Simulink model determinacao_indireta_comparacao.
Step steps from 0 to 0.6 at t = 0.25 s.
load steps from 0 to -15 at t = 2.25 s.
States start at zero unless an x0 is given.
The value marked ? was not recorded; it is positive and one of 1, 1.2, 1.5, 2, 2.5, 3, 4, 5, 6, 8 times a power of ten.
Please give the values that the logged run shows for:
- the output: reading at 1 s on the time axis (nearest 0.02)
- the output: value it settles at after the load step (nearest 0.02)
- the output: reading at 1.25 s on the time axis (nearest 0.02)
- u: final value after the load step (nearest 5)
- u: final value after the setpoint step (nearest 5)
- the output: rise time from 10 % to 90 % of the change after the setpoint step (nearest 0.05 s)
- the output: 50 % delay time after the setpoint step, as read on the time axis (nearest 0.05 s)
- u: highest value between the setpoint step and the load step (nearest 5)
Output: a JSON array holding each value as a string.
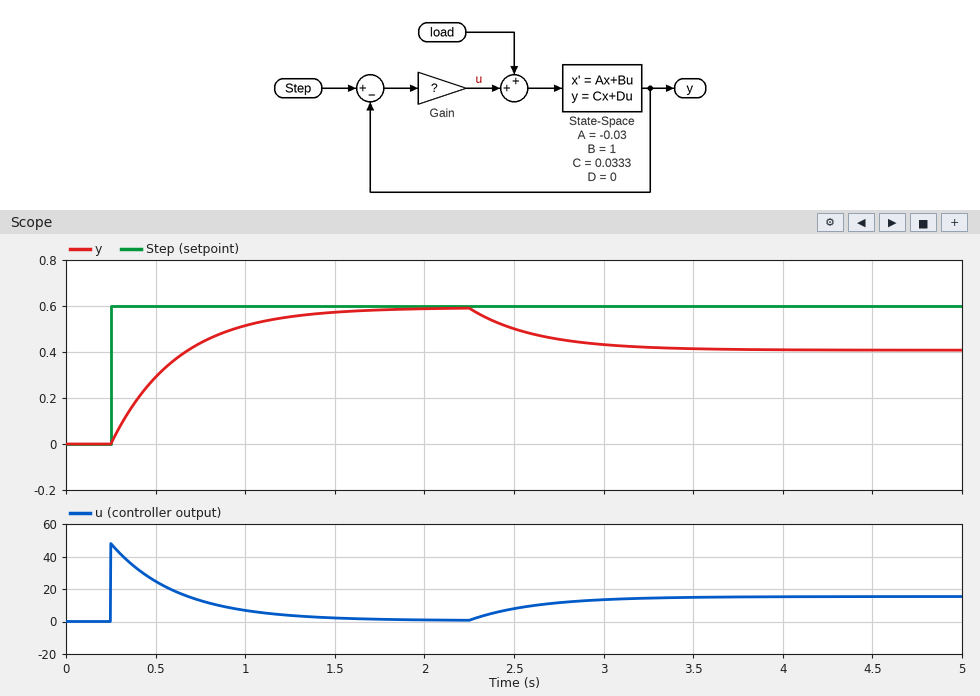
["0.52", "0.40", "0.56", "15", "0", "0.80 s", "0.50 s", "50"]
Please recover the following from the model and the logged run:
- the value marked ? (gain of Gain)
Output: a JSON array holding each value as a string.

["80"]
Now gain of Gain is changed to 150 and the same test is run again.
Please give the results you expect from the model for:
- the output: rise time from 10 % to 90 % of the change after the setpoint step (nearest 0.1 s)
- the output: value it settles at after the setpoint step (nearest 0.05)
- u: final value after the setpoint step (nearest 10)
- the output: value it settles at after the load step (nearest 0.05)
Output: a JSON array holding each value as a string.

["0.4 s", "0.60", "0", "0.50"]
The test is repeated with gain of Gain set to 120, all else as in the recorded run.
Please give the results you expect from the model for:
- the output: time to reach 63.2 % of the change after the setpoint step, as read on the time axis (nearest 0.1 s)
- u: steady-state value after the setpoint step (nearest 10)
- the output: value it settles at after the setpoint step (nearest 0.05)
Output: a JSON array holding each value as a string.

["0.5 s", "0", "0.60"]
